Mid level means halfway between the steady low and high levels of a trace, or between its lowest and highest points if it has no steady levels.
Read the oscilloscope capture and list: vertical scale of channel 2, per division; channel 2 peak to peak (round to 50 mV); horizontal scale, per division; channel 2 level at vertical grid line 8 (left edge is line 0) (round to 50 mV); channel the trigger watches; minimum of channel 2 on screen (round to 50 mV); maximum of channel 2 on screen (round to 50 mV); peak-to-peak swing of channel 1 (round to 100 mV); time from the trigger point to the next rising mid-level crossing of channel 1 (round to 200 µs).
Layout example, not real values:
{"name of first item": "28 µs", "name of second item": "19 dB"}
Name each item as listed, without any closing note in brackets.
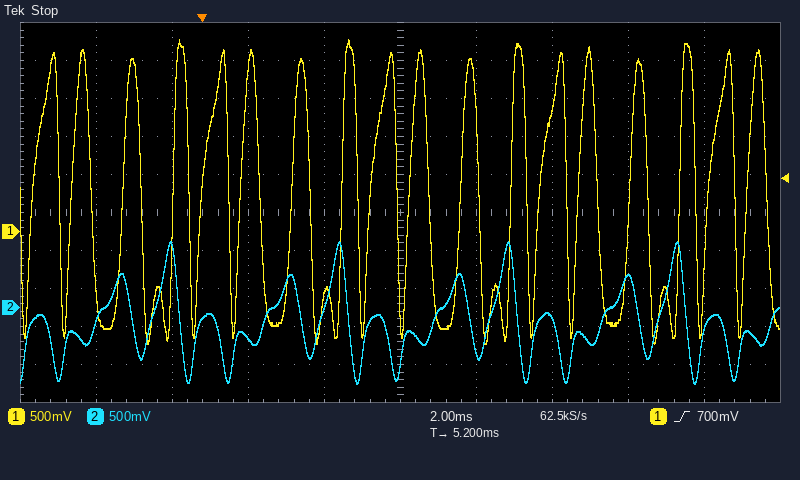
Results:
{"vertical scale of channel 2, per division": "500 mV", "channel 2 peak to peak": "1.85 V", "horizontal scale, per division": "2 ms", "channel 2 level at vertical grid line 8 (left edge is line 0)": "400 mV", "channel the trigger watches": "channel 1", "minimum of channel 2 on screen": "-1.00 V", "maximum of channel 2 on screen": "850 mV", "peak-to-peak swing of channel 1": "4.00 V", "time from the trigger point to the next rising mid-level crossing of channel 1": "1.0 ms"}
